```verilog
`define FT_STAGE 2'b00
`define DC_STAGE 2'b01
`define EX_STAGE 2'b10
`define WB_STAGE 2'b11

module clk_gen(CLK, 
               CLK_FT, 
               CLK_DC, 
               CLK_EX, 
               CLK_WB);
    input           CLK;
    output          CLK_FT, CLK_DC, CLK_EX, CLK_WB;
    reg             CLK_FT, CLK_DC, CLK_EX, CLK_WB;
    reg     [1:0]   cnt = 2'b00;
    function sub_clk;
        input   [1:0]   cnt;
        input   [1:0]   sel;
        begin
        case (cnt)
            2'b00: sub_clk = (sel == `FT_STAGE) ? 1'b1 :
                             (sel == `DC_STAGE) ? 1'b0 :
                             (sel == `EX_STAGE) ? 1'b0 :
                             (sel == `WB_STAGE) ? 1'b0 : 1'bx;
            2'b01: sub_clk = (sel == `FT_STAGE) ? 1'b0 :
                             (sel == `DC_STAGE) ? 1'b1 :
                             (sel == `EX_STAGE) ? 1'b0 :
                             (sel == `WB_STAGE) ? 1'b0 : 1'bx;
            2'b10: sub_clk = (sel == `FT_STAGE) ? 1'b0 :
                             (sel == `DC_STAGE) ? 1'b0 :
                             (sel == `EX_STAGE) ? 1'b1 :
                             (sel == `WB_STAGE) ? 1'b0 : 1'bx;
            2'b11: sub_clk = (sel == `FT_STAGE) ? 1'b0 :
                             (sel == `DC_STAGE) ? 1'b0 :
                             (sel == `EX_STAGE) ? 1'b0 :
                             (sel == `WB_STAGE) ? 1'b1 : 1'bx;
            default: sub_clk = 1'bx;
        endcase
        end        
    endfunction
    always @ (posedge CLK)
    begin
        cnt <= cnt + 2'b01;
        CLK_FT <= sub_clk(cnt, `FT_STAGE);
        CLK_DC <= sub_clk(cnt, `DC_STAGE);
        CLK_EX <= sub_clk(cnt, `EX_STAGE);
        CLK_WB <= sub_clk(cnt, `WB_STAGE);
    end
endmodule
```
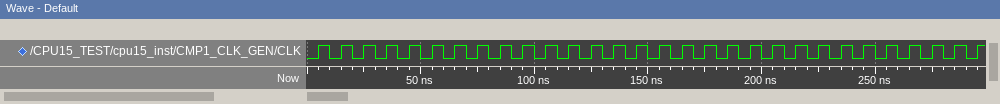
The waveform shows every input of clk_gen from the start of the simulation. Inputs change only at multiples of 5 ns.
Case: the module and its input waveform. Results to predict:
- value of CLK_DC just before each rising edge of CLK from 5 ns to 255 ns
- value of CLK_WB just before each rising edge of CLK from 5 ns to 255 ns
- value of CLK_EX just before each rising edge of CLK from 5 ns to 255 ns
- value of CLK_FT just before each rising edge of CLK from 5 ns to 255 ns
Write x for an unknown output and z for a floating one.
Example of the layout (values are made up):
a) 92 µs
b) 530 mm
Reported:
a) x 0 1 0 0 0 1 0 0 0 1 0 0 0 1 0 0 0 1 0 0 0 1 0 0 0
b) x 0 0 0 1 0 0 0 1 0 0 0 1 0 0 0 1 0 0 0 1 0 0 0 1 0
c) x 0 0 1 0 0 0 1 0 0 0 1 0 0 0 1 0 0 0 1 0 0 0 1 0 0
d) x 1 0 0 0 1 0 0 0 1 0 0 0 1 0 0 0 1 0 0 0 1 0 0 0 1
